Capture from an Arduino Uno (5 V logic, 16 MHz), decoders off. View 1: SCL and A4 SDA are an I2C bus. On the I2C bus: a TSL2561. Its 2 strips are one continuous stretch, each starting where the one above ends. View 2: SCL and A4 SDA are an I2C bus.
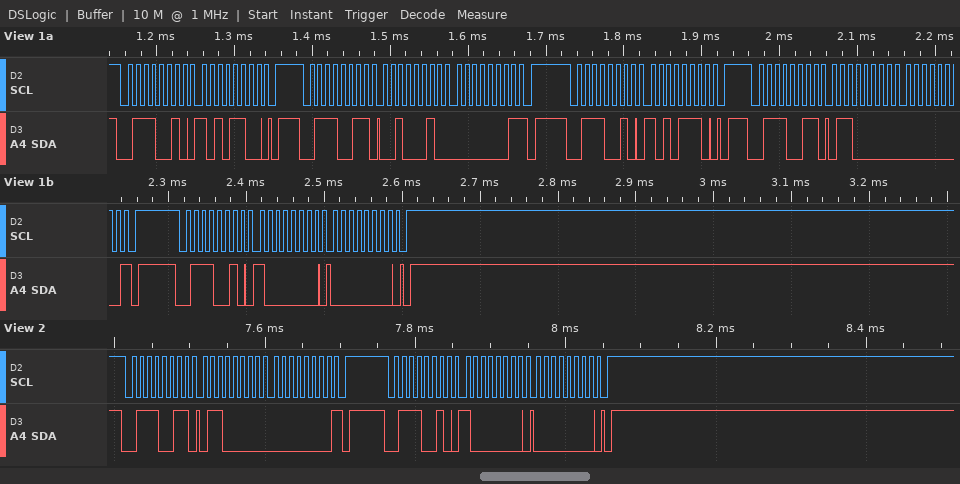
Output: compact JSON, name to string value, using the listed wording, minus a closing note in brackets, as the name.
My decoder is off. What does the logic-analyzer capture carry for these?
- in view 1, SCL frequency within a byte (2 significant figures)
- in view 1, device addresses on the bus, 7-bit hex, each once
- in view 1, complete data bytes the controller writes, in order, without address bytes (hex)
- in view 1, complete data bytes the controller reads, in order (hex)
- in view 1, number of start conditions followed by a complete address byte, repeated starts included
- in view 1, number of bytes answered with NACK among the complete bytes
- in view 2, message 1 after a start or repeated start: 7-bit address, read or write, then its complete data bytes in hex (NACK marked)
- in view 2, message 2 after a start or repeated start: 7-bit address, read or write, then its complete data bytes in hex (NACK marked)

{"in view 1, SCL frequency within a byte": "100 kHz", "in view 1, device addresses on the bus, 7-bit hex, each once": "0x39", "in view 1, complete data bytes the controller writes, in order, without address bytes": "AC AE 80 00", "in view 1, complete data bytes the controller reads, in order": "22 01 60 00", "in view 1, number of start conditions followed by a complete address byte, repeated starts included": "5", "in view 1, number of bytes answered with NACK among the complete bytes": "2", "in view 2, message 1 after a start or repeated start: 7-bit address, read or write, then its complete data bytes in hex": "0x39 read: 60 00 NACK", "in view 2, message 2 after a start or repeated start: 7-bit address, read or write, then its complete data bytes in hex": "0x39 write: 80 00"}
